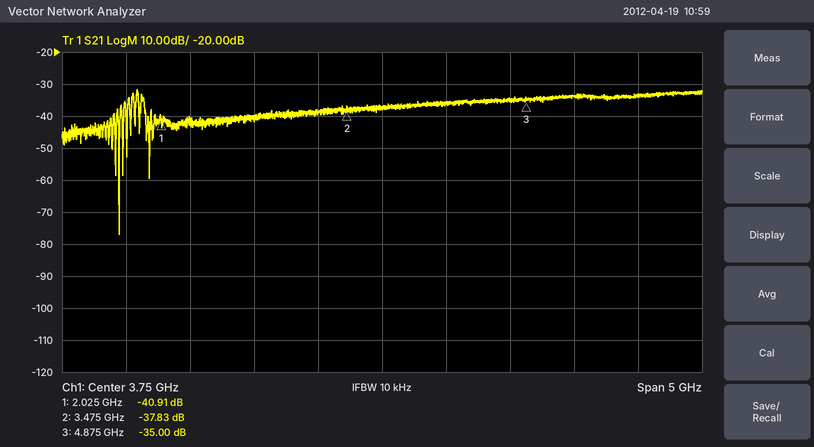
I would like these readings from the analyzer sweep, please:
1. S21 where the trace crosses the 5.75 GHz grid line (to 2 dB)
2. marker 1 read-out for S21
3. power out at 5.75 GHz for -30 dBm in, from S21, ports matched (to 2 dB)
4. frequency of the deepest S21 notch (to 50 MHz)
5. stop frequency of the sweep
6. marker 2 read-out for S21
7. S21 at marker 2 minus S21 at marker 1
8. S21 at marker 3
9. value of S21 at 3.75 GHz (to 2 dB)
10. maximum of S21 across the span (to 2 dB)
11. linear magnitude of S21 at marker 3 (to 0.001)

-34 dB
-40.91 dB
-64 dBm
1.70 GHz
6.25 GHz
-37.83 dB
3.08 dB
-35.00 dB
-38 dB
-32 dB
0.018
